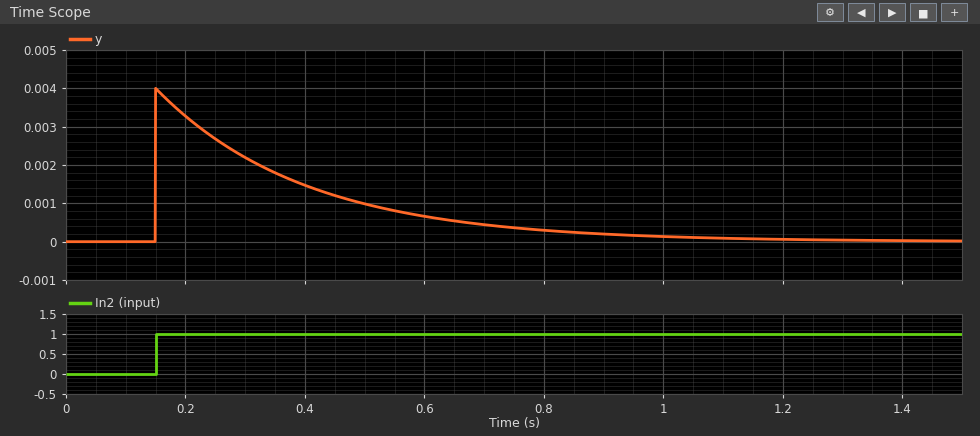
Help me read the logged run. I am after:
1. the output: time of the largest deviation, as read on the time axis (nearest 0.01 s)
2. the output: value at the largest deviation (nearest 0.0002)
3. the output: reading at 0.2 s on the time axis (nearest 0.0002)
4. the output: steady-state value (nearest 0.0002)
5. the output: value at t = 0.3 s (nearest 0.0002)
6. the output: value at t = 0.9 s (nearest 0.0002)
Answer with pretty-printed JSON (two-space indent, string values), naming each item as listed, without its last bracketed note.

{
  "the output: time of the largest deviation, as read on the time axis": "0.15 s",
  "the output: value at the largest deviation": "0.0040",
  "the output: reading at 0.2 s on the time axis": "0.0032",
  "the output: steady-state value": "0.0000",
  "the output: value at t = 0.3 s": "0.0022",
  "the output: value at t = 0.9 s": "0.0002"
}
